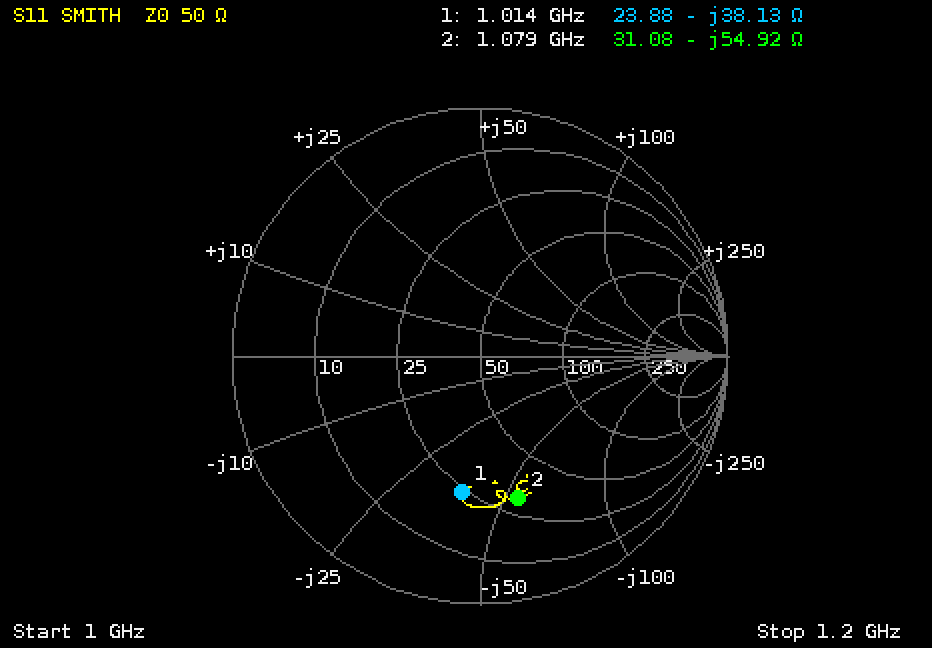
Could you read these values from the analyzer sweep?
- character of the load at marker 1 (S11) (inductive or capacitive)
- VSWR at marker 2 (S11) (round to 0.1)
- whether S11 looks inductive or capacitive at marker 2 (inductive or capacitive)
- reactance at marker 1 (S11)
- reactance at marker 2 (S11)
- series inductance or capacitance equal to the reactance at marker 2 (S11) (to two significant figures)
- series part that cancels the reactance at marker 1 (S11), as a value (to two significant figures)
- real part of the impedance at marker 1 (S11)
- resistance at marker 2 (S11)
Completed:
capacitive
3.9
capacitive
-38.13 Ω
-54.92 Ω
2.7 pF
6.0 nH
23.88 Ω
31.08 Ω
